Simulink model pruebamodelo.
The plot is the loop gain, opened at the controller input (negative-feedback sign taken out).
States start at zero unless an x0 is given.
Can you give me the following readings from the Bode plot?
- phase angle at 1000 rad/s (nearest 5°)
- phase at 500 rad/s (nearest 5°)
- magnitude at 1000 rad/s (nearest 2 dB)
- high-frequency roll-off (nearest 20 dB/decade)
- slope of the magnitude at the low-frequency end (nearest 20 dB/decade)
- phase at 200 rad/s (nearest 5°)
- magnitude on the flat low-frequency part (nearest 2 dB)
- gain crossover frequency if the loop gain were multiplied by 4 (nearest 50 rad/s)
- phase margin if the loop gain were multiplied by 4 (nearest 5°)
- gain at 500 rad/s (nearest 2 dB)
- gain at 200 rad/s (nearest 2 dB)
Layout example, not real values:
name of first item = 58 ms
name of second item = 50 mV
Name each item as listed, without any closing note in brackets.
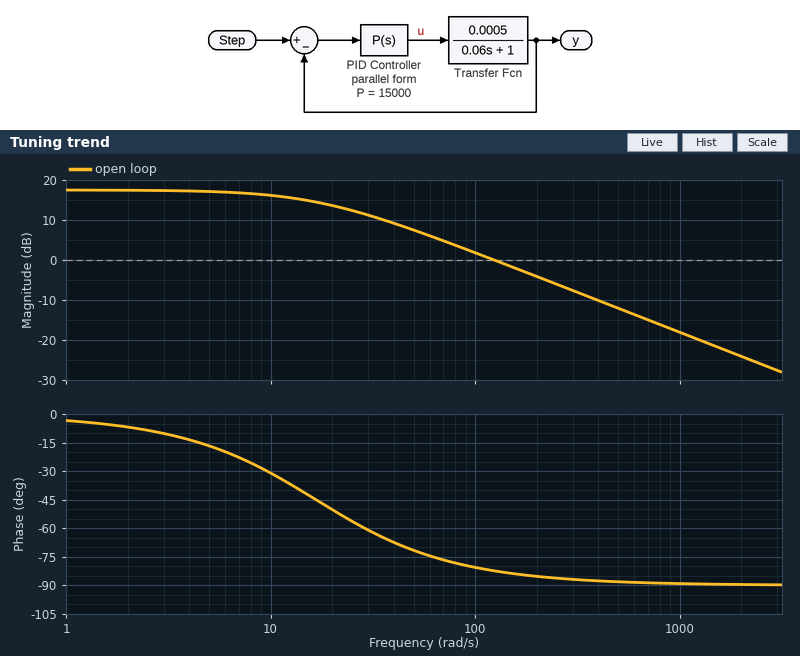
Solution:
phase angle at 1000 rad/s = -90°
phase at 500 rad/s = -90°
magnitude at 1000 rad/s = -18 dB
high-frequency roll-off = -20 dB/decade
slope of the magnitude at the low-frequency end = 0 dB/decade
phase at 200 rad/s = -85°
magnitude on the flat low-frequency part = 18 dB
gain crossover frequency if the loop gain were multiplied by 4 = 500 rad/s
phase margin if the loop gain were multiplied by 4 = 90°
gain at 500 rad/s = -12 dB
gain at 200 rad/s = -4 dB
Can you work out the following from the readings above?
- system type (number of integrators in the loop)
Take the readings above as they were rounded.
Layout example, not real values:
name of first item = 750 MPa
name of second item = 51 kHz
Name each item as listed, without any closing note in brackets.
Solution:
system type = 0
